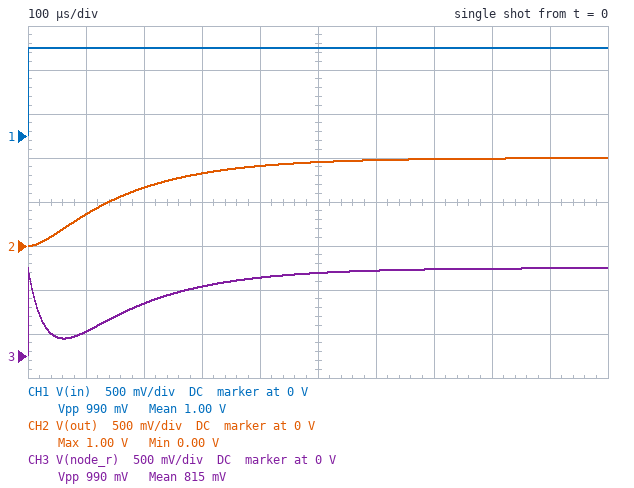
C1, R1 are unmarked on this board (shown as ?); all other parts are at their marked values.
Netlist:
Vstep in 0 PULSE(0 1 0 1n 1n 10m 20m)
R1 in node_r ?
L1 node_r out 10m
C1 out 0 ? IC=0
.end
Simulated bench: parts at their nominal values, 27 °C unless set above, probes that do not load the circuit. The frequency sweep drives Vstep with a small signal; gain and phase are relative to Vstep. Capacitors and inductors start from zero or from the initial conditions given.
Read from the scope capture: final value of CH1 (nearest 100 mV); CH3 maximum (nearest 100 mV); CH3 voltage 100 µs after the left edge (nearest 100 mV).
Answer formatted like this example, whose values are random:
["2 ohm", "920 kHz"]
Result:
["1.0 V", "1.0 V", "300 mV"]
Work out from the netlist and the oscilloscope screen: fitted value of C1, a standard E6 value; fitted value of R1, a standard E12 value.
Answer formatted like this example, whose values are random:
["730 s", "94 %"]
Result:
["470 nF", "390 Ω"]
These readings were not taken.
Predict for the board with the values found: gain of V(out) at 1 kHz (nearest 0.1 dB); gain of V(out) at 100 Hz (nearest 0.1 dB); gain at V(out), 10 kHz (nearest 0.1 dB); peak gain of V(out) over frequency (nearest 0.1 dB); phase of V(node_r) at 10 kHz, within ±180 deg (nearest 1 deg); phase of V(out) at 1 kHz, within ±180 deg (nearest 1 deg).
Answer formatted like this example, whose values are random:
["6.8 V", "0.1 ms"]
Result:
["-3.0 dB", "0 dB", "-26.4 dB", "0 dB", "33 deg", "-55 deg"]
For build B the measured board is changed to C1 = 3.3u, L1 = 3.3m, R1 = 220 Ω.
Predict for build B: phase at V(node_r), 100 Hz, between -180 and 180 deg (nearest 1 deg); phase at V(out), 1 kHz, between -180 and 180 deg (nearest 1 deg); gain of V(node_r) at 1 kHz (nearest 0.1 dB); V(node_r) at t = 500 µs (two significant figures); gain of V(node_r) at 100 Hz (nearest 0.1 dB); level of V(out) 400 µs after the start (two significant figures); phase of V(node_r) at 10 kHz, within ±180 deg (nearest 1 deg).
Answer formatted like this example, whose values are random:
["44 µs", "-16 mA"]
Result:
["-25 deg", "-83 deg", "-18.1 dB", "480 mV", "-0.8 dB", "420 mV", "47 deg"]
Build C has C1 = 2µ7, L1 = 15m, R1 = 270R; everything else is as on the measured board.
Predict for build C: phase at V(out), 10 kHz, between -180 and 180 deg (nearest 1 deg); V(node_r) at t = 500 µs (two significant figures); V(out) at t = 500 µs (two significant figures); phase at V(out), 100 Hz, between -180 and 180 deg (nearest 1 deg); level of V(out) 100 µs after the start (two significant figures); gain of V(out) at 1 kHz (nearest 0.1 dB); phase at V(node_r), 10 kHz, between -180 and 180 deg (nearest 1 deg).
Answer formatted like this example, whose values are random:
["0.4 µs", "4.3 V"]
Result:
["-164 deg", "430 mV", "480 mV", "-25 deg", "72 mV", "-13.3 dB", "16 deg"]
